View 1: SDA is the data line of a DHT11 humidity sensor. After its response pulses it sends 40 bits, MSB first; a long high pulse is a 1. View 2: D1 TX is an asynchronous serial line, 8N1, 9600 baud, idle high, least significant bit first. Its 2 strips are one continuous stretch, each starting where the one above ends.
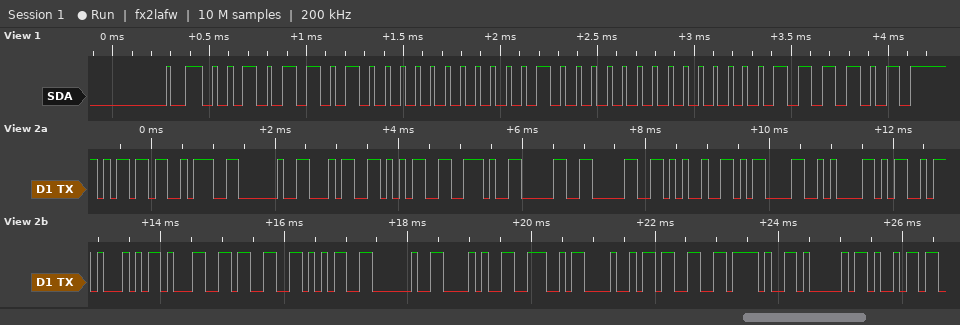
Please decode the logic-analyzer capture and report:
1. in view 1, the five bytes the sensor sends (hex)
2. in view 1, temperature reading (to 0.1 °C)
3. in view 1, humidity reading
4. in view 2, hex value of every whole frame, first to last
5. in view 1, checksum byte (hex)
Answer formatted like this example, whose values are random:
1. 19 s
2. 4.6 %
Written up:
1. 2D 00 10 00 3D
2. 16.0 °C
3. 45 %
4. 0x6D 0x3A 0x20 0x34 0x35 0x2E 0x30 0x30 0x25 0x0D 0x0A 0x4D 0x51 0x31 0x33 0x35 0x20 0x28 0x4E 0x48 0x33 0x2F 0x41 0x69
5. 0x3D
